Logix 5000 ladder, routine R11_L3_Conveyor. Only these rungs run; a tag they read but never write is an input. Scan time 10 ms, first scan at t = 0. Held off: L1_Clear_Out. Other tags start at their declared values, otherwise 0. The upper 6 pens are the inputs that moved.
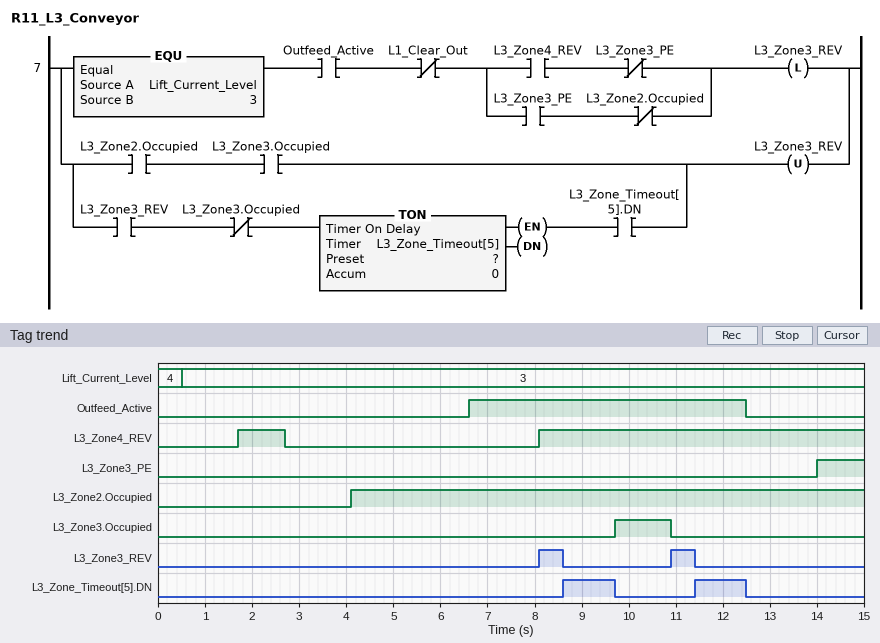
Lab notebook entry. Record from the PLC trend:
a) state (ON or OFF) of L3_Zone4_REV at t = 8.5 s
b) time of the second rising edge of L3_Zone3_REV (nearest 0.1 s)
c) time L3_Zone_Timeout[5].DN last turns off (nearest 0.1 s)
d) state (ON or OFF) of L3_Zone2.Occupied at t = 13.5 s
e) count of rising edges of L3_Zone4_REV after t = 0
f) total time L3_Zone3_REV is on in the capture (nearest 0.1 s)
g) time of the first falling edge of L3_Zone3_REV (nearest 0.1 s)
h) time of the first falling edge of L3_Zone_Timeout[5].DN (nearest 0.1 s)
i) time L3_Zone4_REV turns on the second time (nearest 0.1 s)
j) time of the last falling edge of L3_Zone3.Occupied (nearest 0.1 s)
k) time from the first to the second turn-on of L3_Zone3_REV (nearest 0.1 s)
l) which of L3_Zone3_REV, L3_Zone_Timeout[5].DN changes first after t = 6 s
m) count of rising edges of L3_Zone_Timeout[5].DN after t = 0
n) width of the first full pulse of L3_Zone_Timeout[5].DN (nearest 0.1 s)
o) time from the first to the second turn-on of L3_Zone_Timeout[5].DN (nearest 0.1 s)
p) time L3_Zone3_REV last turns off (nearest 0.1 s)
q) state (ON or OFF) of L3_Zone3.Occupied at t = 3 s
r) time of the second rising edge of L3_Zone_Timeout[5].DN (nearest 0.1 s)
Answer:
ON
10.9 s
12.5 s
ON
2
1.0 s
8.6 s
9.7 s
8.1 s
10.9 s
2.8 s
L3_Zone3_REV
2
1.1 s
2.8 s
11.4 s
OFF
11.4 s
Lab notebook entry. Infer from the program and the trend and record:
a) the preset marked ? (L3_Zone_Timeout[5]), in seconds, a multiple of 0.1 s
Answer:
0.5 s
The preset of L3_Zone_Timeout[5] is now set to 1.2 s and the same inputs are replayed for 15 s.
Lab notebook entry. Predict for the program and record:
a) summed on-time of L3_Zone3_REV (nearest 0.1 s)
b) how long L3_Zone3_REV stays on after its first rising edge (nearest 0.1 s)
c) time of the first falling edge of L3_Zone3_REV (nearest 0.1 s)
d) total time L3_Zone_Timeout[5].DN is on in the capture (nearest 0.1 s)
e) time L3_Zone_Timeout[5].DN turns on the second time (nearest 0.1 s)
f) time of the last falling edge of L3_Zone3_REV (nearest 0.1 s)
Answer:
2.4 s
1.2 s
9.3 s
0.8 s
12.1 s
12.1 s
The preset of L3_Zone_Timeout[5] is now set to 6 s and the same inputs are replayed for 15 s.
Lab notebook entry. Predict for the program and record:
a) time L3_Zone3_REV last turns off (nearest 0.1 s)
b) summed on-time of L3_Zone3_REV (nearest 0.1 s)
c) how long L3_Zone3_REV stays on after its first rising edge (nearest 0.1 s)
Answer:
9.7 s
5.7 s
1.6 s
